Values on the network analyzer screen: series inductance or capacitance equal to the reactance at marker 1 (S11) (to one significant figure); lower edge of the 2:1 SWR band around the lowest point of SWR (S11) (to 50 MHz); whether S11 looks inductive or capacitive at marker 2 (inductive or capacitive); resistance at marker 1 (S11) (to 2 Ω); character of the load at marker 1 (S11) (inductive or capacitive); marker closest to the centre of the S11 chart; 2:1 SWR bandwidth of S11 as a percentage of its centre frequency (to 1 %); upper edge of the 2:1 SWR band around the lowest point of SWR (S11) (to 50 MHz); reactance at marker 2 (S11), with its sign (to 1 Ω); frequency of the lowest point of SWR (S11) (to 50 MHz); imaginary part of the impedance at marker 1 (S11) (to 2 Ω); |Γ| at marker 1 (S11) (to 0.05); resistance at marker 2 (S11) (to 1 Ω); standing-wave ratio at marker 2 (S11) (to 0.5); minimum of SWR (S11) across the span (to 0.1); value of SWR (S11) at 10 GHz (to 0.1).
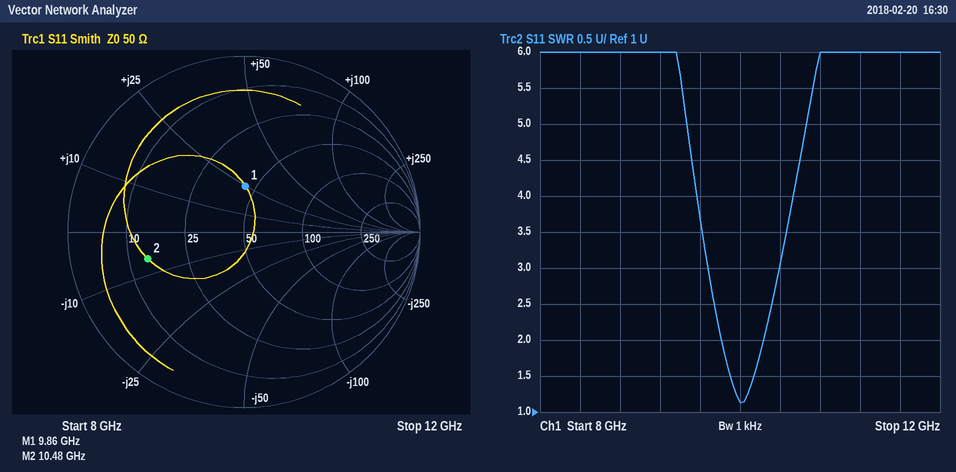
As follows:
400 pH
9.80 GHz
capacitive
44 Ω
inductive
marker 1
4 %
10.25 GHz
-6 Ω
10.00 GHz
+24 Ω
0.25
14 Ω
3.5
1.1
1.1
